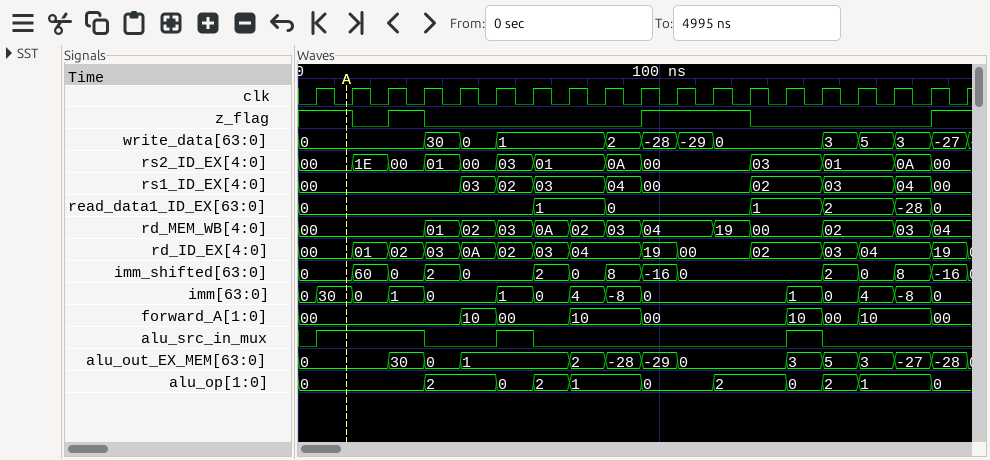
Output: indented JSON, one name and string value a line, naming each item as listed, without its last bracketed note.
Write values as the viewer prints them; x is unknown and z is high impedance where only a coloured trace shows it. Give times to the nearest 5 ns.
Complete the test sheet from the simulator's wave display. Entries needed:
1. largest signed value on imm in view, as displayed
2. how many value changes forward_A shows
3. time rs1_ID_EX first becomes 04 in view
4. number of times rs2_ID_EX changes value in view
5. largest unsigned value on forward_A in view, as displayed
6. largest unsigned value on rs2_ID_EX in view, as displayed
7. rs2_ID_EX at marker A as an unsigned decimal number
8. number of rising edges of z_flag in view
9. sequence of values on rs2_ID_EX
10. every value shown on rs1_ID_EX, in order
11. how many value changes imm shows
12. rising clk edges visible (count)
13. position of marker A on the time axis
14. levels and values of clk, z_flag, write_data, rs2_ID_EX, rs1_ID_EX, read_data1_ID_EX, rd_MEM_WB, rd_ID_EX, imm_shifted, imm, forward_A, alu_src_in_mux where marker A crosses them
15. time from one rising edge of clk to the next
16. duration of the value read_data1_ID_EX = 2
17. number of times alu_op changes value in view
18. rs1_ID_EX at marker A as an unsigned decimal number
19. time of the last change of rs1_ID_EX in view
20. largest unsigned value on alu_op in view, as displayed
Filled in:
{
  "largest signed value on imm in view, as displayed": "30",
  "how many value changes forward_A shows": "8",
  "time rs1_ID_EX first becomes 04 in view": "85 ns",
  "number of times rs2_ID_EX changes value in view": "12",
  "largest unsigned value on forward_A in view, as displayed": "10",
  "largest unsigned value on rs2_ID_EX in view, as displayed": "1E",
  "rs2_ID_EX at marker A as an unsigned decimal number": "0",
  "number of rising edges of z_flag in view": "3",
  "sequence of values on rs2_ID_EX": "00, 1E, 00, 01, 00, 03, 01, 0A, 00, 03, 01, 0A, 00",
  "every value shown on rs1_ID_EX, in order": "00, 03, 02, 03, 04, 00, 02, 03, 04, 00",
  "how many value changes imm shows": "14",
  "rising clk edges visible": "19",
  "position of marker A on the time axis": "15 ns",
  "levels and values of clk, z_flag, write_data, rs2_ID_EX, rs1_ID_EX, read_data1_ID_EX, rd_MEM_WB, rd_ID_EX, imm_shifted, imm, forward_A, alu_src_in_mux where marker A crosses them": "clk=0, z_flag=1, write_data=0, rs2_ID_EX=00, rs1_ID_EX=00, read_data1_ID_EX=0, rd_MEM_WB=00, rd_ID_EX=00, imm_shifted=0, imm=30, forward_A=00, alu_src_in_mux=1",
  "time from one rising edge of clk to the next": "10 ns",
  "duration of the value read_data1_ID_EX = 2": "20 ns",
  "number of times alu_op changes value in view": "10",
  "rs1_ID_EX at marker A as an unsigned decimal number": "0",
  "time of the last change of rs1_ID_EX in view": "175 ns",
  "largest unsigned value on alu_op in view, as displayed": "2"
}
